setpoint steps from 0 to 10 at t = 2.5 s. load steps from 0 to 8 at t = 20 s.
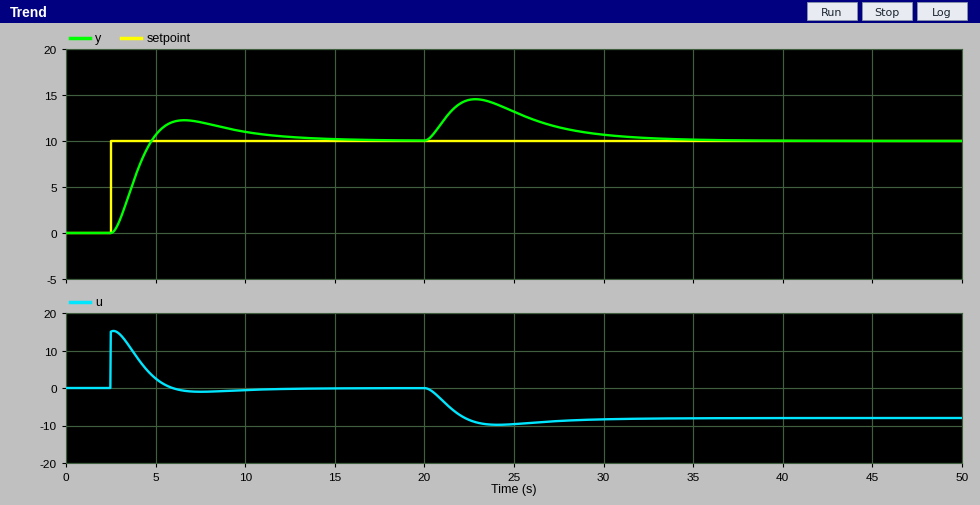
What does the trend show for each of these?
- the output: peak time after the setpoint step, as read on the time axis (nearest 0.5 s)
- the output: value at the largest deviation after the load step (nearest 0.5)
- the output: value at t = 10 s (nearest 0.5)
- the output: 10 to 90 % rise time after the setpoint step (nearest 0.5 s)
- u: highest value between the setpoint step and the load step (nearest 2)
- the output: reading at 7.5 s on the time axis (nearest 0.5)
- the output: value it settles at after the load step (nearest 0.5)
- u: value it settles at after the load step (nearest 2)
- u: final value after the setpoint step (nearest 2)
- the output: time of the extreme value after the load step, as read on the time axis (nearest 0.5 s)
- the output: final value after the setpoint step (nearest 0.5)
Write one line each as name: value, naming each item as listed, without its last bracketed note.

the output: peak time after the setpoint step, as read on the time axis: 6.5 s
the output: value at the largest deviation after the load step: 14.5
the output: value at t = 10 s: 11.0
the output: 10 to 90 % rise time after the setpoint step: 1.5 s
u: highest value between the setpoint step and the load step: 16
the output: reading at 7.5 s on the time axis: 12.0
the output: value it settles at after the load step: 10.0
u: value it settles at after the load step: -8
u: final value after the setpoint step: 0
the output: time of the extreme value after the load step, as read on the time axis: 23.0 s
the output: final value after the setpoint step: 10.0
